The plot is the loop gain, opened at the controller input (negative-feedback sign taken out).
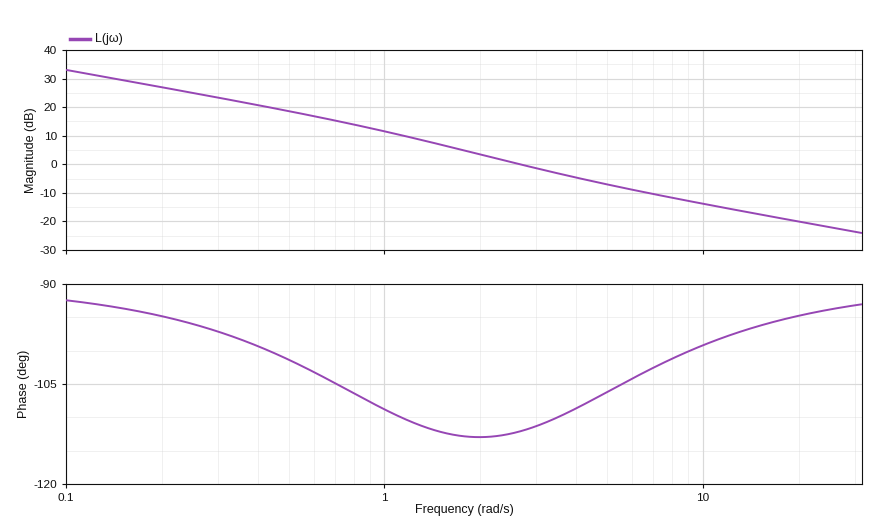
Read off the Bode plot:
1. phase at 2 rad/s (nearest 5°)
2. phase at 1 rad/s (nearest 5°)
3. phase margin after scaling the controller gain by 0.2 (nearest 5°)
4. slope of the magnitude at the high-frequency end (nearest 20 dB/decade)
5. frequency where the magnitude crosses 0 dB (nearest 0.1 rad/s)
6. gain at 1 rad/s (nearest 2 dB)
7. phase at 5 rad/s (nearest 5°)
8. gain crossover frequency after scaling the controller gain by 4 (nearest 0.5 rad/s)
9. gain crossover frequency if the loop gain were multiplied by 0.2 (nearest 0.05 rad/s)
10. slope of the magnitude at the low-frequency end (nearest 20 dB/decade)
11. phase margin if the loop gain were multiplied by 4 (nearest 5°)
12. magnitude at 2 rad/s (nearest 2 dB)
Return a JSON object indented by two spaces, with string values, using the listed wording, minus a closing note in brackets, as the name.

{
  "phase at 2 rad/s": "-115°",
  "phase at 1 rad/s": "-110°",
  "phase margin after scaling the controller gain by 0.2": "75°",
  "slope of the magnitude at the high-frequency end": "-20 dB/decade",
  "frequency where the magnitude crosses 0 dB": "2.7 rad/s",
  "gain at 1 rad/s": "12 dB",
  "phase at 5 rad/s": "-105°",
  "gain crossover frequency after scaling the controller gain by 4": "8.5 rad/s",
  "gain crossover frequency if the loop gain were multiplied by 0.2": "0.80 rad/s",
  "slope of the magnitude at the low-frequency end": "-20 dB/decade",
  "phase margin if the loop gain were multiplied by 4": "80°",
  "magnitude at 2 rad/s": "4 dB"
}
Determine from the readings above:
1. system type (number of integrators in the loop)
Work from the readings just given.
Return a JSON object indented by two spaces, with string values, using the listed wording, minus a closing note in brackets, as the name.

{
  "system type": "1"
}
